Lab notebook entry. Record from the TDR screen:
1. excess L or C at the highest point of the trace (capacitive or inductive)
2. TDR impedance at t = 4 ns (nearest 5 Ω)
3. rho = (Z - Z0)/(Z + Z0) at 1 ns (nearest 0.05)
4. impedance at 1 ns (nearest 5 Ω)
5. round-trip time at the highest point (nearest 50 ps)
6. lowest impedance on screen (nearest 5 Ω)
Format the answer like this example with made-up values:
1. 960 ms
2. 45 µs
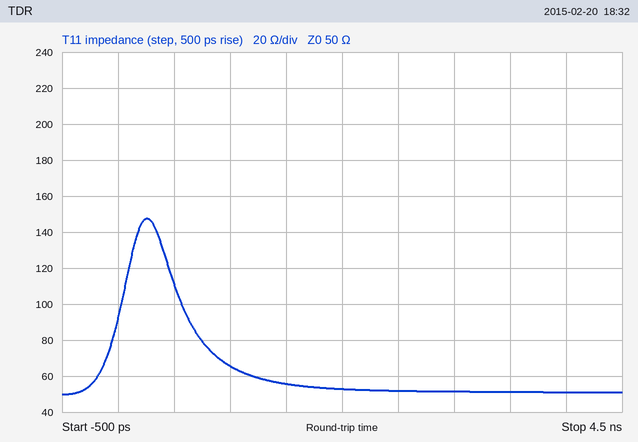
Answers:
1. inductive
2. 50 Ω
3. +0.15
4. 65 Ω
5. 250 ps
6. 50 Ω
